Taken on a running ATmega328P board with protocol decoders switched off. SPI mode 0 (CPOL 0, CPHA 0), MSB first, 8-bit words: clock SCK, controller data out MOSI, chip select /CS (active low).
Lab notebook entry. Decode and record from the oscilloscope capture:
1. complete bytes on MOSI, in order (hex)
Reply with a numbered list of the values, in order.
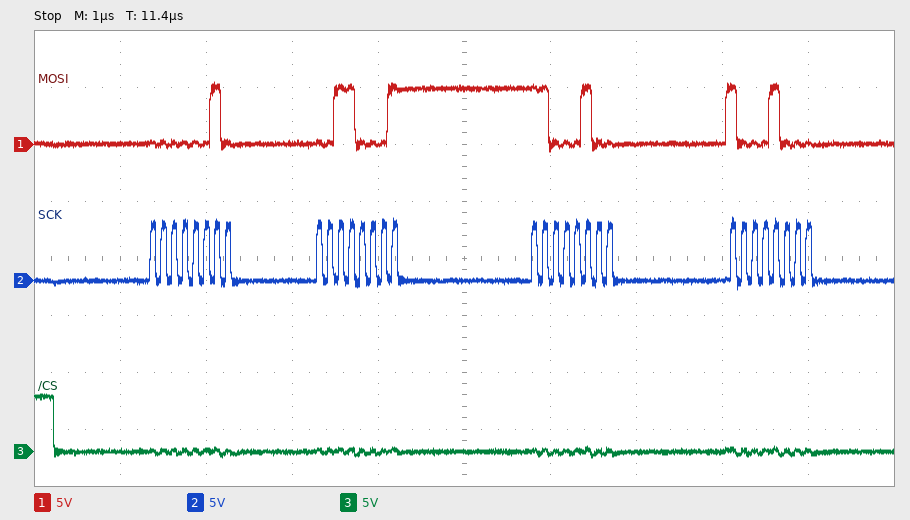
1. 02 31 C4 88
